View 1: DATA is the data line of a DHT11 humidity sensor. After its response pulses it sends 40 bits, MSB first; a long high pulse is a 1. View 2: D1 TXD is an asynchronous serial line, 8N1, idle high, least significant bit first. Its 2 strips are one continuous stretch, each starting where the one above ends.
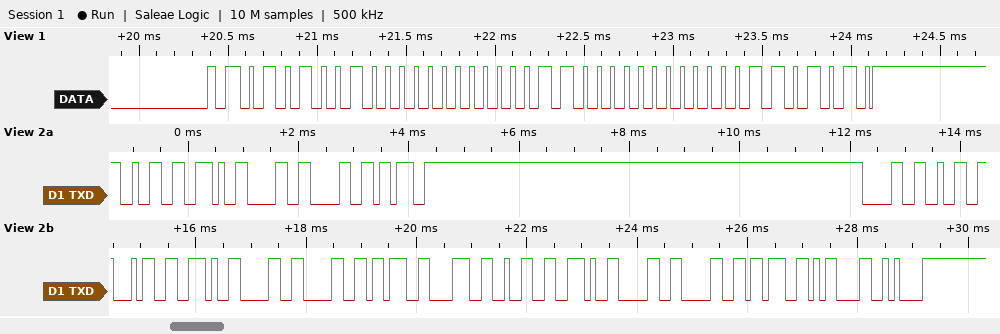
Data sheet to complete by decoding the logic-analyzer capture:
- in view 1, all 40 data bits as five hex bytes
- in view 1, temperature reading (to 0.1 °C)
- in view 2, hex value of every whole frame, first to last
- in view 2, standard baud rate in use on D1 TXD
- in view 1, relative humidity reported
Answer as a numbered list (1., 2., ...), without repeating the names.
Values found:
1. 52 00 18 00 6A
2. 24.0 °C
3. 32 2E 30 30 3B 30 32 34 2E 30 30 3B 38 32 2E 30 30 3B 0D 0A
4. 9600 baud
5. 82 %
